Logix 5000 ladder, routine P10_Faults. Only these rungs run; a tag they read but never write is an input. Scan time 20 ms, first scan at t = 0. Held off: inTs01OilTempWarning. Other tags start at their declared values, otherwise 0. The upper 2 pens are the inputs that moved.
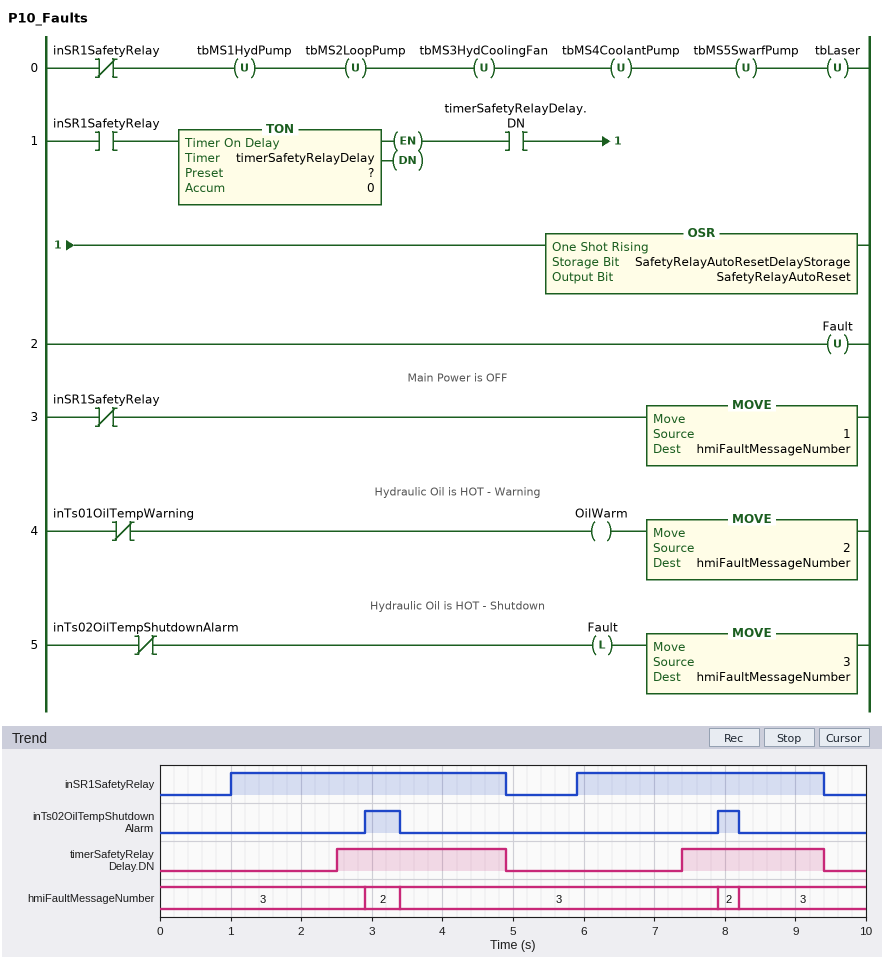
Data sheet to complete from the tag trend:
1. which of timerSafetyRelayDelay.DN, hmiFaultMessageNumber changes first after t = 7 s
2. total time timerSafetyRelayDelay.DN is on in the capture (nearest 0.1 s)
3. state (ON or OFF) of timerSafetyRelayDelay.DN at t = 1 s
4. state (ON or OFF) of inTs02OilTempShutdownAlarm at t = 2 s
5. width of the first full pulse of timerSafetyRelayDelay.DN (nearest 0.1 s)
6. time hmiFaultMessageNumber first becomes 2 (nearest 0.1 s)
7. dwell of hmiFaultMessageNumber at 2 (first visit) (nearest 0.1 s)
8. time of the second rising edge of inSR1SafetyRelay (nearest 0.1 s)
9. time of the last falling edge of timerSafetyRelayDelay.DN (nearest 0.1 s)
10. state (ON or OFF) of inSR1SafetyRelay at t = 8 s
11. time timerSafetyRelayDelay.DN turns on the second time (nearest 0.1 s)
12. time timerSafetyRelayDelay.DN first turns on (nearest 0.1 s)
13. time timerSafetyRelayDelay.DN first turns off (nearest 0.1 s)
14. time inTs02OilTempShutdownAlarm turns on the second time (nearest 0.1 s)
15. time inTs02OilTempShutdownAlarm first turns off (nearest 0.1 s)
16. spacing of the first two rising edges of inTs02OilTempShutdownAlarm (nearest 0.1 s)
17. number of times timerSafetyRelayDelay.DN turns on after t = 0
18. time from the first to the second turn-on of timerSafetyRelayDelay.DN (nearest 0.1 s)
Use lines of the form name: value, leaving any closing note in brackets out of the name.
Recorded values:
which of timerSafetyRelayDelay.DN, hmiFaultMessageNumber changes first after t = 7 s: timerSafetyRelayDelay.DN
total time timerSafetyRelayDelay.DN is on in the capture: 4.4 s
state (ON or OFF) of timerSafetyRelayDelay.DN at t = 1 s: OFF
state (ON or OFF) of inTs02OilTempShutdownAlarm at t = 2 s: OFF
width of the first full pulse of timerSafetyRelayDelay.DN: 2.4 s
time hmiFaultMessageNumber first becomes 2: 2.9 s
dwell of hmiFaultMessageNumber at 2 (first visit): 0.5 s
time of the second rising edge of inSR1SafetyRelay: 5.9 s
time of the last falling edge of timerSafetyRelayDelay.DN: 9.4 s
state (ON or OFF) of inSR1SafetyRelay at t = 8 s: ON
time timerSafetyRelayDelay.DN turns on the second time: 7.4 s
time timerSafetyRelayDelay.DN first turns on: 2.5 s
time timerSafetyRelayDelay.DN first turns off: 4.9 s
time inTs02OilTempShutdownAlarm turns on the second time: 7.9 s
time inTs02OilTempShutdownAlarm first turns off: 3.4 s
spacing of the first two rising edges of inTs02OilTempShutdownAlarm: 5.0 s
number of times timerSafetyRelayDelay.DN turns on after t = 0: 2
time from the first to the second turn-on of timerSafetyRelayDelay.DN: 4.9 s
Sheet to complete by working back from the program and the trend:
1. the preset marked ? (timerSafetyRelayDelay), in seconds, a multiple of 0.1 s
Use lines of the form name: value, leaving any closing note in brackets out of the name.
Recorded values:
the preset marked ? (timerSafetyRelayDelay), in seconds, a multiple of 0.1 s: 1.5 s
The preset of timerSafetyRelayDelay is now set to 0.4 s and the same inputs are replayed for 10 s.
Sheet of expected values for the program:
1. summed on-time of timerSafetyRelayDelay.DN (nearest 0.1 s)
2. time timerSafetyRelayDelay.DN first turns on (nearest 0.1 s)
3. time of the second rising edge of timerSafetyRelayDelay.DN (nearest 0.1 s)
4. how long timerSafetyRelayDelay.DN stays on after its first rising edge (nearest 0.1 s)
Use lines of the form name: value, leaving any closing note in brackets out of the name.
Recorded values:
summed on-time of timerSafetyRelayDelay.DN: 6.6 s
time timerSafetyRelayDelay.DN first turns on: 1.4 s
time of the second rising edge of timerSafetyRelayDelay.DN: 6.3 s
how long timerSafetyRelayDelay.DN stays on after its first rising edge: 3.5 s
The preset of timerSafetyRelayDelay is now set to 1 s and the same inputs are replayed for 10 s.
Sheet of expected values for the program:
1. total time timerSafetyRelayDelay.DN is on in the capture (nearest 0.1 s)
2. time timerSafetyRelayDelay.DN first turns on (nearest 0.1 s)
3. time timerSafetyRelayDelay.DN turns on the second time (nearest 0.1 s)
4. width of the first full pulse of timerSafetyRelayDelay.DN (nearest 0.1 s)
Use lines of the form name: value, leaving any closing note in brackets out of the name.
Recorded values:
total time timerSafetyRelayDelay.DN is on in the capture: 5.4 s
time timerSafetyRelayDelay.DN first turns on: 2.0 s
time timerSafetyRelayDelay.DN turns on the second time: 6.9 s
width of the first full pulse of timerSafetyRelayDelay.DN: 2.9 s
